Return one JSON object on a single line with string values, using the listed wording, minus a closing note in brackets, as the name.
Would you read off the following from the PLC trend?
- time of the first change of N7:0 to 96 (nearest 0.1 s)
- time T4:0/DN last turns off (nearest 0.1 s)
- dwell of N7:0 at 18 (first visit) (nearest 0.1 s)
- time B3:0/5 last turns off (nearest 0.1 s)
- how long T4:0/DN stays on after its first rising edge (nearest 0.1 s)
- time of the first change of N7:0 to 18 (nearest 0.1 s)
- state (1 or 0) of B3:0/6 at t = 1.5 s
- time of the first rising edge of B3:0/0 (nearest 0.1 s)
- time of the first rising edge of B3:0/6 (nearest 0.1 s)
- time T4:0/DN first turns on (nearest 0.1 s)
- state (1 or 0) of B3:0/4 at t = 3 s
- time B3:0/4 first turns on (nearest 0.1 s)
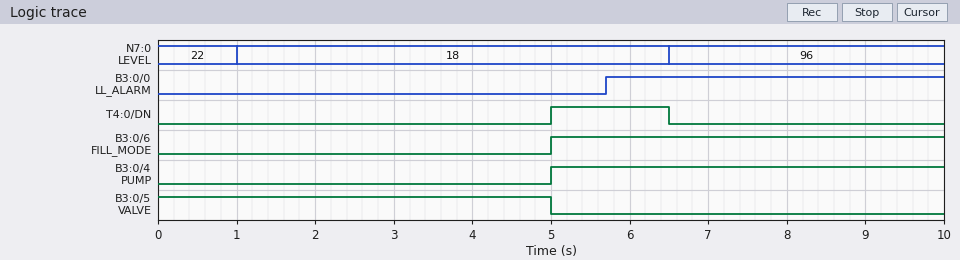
{"time of the first change of N7:0 to 96": "6.5 s", "time T4:0/DN last turns off": "6.5 s", "dwell of N7:0 at 18 (first visit)": "5.5 s", "time B3:0/5 last turns off": "5.0 s", "how long T4:0/DN stays on after its first rising edge": "1.5 s", "time of the first change of N7:0 to 18": "1.0 s", "state (1 or 0) of B3:0/6 at t = 1.5 s": "0", "time of the first rising edge of B3:0/0": "5.7 s", "time of the first rising edge of B3:0/6": "5.0 s", "time T4:0/DN first turns on": "5.0 s", "state (1 or 0) of B3:0/4 at t = 3 s": "0", "time B3:0/4 first turns on": "5.0 s"}
